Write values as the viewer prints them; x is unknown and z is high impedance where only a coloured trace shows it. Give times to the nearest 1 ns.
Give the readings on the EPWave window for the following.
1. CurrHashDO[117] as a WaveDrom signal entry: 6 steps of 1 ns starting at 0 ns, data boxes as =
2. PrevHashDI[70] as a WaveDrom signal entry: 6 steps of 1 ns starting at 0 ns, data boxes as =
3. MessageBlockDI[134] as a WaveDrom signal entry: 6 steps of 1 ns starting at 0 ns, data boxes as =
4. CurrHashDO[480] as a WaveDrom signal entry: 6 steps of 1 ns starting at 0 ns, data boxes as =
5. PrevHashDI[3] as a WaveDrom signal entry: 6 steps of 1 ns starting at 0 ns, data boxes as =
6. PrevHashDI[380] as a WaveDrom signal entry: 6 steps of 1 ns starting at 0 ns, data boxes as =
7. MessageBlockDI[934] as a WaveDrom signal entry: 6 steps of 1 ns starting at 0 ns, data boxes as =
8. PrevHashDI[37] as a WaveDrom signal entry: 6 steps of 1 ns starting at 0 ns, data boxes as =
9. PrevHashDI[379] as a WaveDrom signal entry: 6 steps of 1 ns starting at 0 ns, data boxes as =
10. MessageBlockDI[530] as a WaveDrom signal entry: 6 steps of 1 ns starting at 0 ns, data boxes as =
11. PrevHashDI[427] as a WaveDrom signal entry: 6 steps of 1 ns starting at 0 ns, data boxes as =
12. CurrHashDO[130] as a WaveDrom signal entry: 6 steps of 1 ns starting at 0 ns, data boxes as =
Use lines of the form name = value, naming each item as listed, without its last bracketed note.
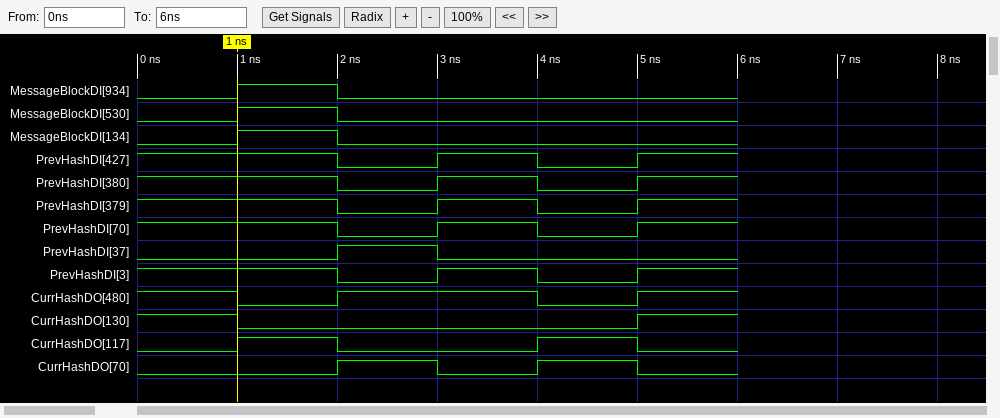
CurrHashDO[117] as a WaveDrom signal entry: 6 steps of 1 ns starting at 0 ns, data boxes as = = {name: 'CurrHashDO[117]', wave: '010.10'}
PrevHashDI[70] as a WaveDrom signal entry: 6 steps of 1 ns starting at 0 ns, data boxes as = = {name: 'PrevHashDI[70]', wave: '1.0101'}
MessageBlockDI[134] as a WaveDrom signal entry: 6 steps of 1 ns starting at 0 ns, data boxes as = = {name: 'MessageBlockDI[134]', wave: '010...'}
CurrHashDO[480] as a WaveDrom signal entry: 6 steps of 1 ns starting at 0 ns, data boxes as = = {name: 'CurrHashDO[480]', wave: '101.01'}
PrevHashDI[3] as a WaveDrom signal entry: 6 steps of 1 ns starting at 0 ns, data boxes as = = {name: 'PrevHashDI[3]', wave: '1.0101'}
PrevHashDI[380] as a WaveDrom signal entry: 6 steps of 1 ns starting at 0 ns, data boxes as = = {name: 'PrevHashDI[380]', wave: '1.0101'}
MessageBlockDI[934] as a WaveDrom signal entry: 6 steps of 1 ns starting at 0 ns, data boxes as = = {name: 'MessageBlockDI[934]', wave: '010...'}
PrevHashDI[37] as a WaveDrom signal entry: 6 steps of 1 ns starting at 0 ns, data boxes as = = {name: 'PrevHashDI[37]', wave: '0.10..'}
PrevHashDI[379] as a WaveDrom signal entry: 6 steps of 1 ns starting at 0 ns, data boxes as = = {name: 'PrevHashDI[379]', wave: '1.0101'}
MessageBlockDI[530] as a WaveDrom signal entry: 6 steps of 1 ns starting at 0 ns, data boxes as = = {name: 'MessageBlockDI[530]', wave: '010...'}
PrevHashDI[427] as a WaveDrom signal entry: 6 steps of 1 ns starting at 0 ns, data boxes as = = {name: 'PrevHashDI[427]', wave: '1.0101'}
CurrHashDO[130] as a WaveDrom signal entry: 6 steps of 1 ns starting at 0 ns, data boxes as = = {name: 'CurrHashDO[130]', wave: '10...1'}
